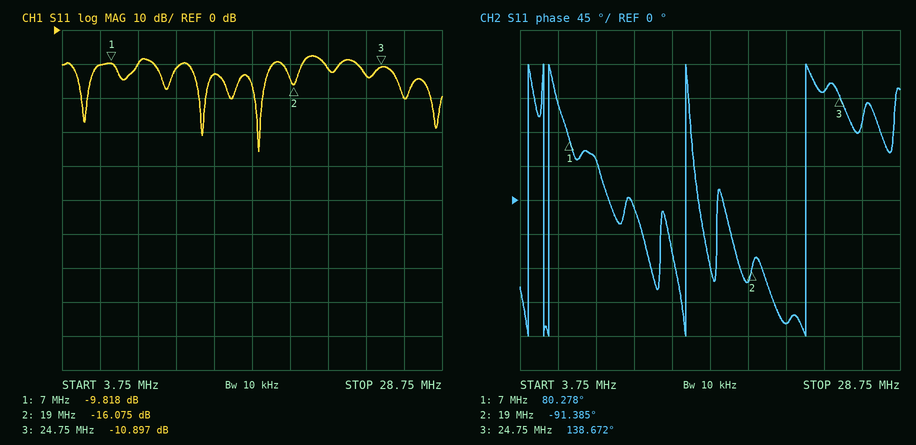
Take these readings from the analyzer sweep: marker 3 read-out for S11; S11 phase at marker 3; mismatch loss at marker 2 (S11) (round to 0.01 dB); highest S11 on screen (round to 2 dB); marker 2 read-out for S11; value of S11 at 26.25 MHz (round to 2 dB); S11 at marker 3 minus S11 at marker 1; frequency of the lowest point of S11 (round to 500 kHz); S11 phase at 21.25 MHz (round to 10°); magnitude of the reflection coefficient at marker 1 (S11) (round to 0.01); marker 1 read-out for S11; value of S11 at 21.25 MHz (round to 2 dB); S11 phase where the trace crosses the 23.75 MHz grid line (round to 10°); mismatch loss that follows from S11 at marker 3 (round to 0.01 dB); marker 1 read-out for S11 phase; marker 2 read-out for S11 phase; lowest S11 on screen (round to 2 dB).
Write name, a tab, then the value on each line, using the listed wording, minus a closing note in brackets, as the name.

marker 3 read-out for S11	-10.897 dB
S11 phase at marker 3	138.672°
mismatch loss at marker 2 (S11)	0.11 dB
highest S11 on screen	-8 dB
marker 2 read-out for S11	-16.075 dB
value of S11 at 26.25 MHz	-20 dB
S11 at marker 3 minus S11 at marker 1	-1.079 dB
frequency of the lowest point of S11	16.5 MHz
S11 phase at 21.25 MHz	-160°
magnitude of the reflection coefficient at marker 1 (S11)	0.32
marker 1 read-out for S11	-9.818 dB
value of S11 at 21.25 MHz	-12 dB
S11 phase where the trace crosses the 23.75 MHz grid line	140°
mismatch loss that follows from S11 at marker 3	0.37 dB
marker 1 read-out for S11 phase	80.278°
marker 2 read-out for S11 phase	-91.385°
lowest S11 on screen	-36 dB
